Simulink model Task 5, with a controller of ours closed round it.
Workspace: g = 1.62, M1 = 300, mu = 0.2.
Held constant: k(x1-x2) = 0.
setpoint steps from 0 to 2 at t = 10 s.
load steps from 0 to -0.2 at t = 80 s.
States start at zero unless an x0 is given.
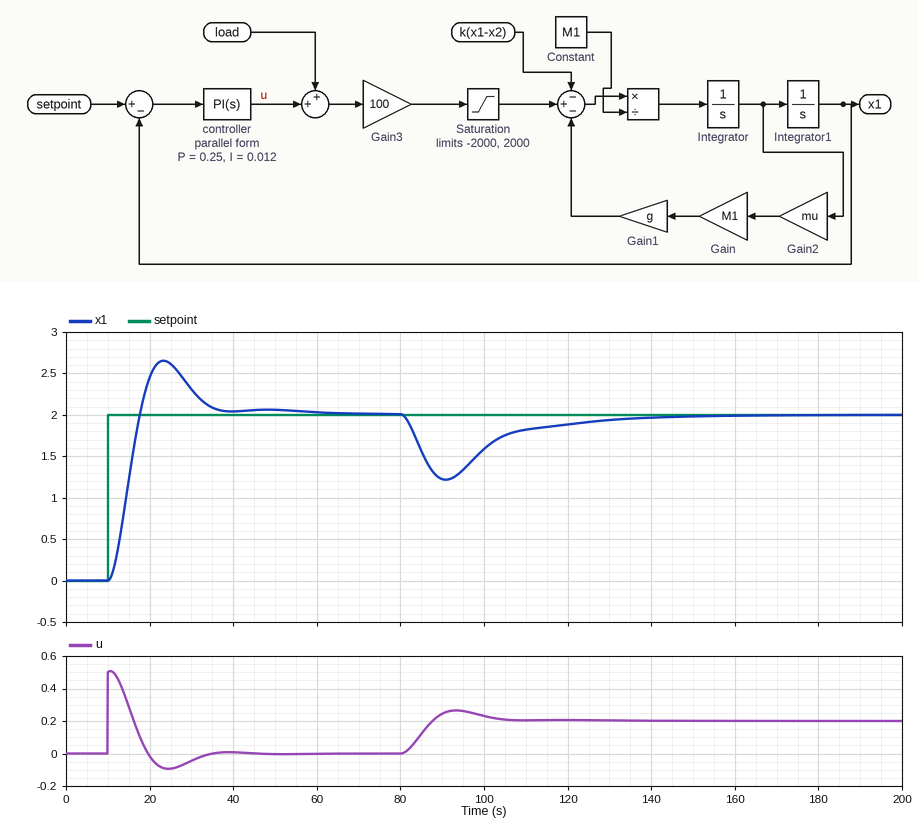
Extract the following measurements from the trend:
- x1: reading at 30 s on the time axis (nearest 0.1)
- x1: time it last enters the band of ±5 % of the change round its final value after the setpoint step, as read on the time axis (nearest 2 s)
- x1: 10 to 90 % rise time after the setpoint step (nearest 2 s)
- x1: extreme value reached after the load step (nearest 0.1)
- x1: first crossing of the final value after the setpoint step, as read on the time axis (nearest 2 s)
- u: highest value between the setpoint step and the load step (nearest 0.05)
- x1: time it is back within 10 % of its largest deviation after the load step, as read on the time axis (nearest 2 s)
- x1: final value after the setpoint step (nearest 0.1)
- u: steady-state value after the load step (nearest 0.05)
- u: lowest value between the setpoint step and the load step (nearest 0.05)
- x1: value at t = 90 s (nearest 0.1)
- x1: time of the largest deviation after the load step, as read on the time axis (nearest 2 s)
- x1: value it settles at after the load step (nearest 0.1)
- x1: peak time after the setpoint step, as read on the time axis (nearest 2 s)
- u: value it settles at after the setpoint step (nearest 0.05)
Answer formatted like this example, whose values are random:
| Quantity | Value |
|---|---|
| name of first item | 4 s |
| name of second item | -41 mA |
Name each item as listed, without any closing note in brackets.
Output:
| Quantity | Value |
|---|---|
| x1: reading at 30 s on the time axis | 2.3 |
| x1: time it last enters the band of ±5 % of the change round its final value after the setpoint step, as read on the time axis | 34 s |
| x1: 10 to 90 % rise time after the setpoint step | 6 s |
| x1: extreme value reached after the load step | 1.2 |
| x1: first crossing of the final value after the setpoint step, as read on the time axis | 18 s |
| u: highest value between the setpoint step and the load step | 0.50 |
| x1: time it is back within 10 % of its largest deviation after the load step, as read on the time axis | 126 s |
| x1: final value after the setpoint step | 2.0 |
| u: steady-state value after the load step | 0.20 |
| u: lowest value between the setpoint step and the load step | -0.10 |
| x1: value at t = 90 s | 1.2 |
| x1: time of the largest deviation after the load step, as read on the time axis | 90 s |
| x1: value it settles at after the load step | 2.0 |
| x1: peak time after the setpoint step, as read on the time axis | 24 s |
| u: value it settles at after the setpoint step | 0.00 |
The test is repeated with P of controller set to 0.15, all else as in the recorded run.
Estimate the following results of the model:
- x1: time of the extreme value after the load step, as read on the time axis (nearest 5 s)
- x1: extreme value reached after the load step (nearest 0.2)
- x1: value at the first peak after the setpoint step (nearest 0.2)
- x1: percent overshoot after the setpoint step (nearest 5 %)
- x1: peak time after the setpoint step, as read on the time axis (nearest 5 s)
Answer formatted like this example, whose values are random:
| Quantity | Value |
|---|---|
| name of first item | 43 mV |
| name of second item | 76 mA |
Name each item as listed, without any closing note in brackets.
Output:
| Quantity | Value |
|---|---|
| x1: time of the extreme value after the load step, as read on the time axis | 95 s |
| x1: extreme value reached after the load step | 1.0 |
| x1: value at the first peak after the setpoint step | 2.8 |
| x1: percent overshoot after the setpoint step | 45 % |
| x1: peak time after the setpoint step, as read on the time axis | 30 s |
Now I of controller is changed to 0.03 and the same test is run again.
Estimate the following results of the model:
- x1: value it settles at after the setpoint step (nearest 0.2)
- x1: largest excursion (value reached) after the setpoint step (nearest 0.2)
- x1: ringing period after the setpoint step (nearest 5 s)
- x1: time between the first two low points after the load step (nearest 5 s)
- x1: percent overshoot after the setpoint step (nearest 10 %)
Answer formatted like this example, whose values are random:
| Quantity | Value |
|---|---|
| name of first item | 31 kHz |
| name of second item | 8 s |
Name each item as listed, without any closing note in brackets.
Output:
| Quantity | Value |
|---|---|
| x1: value it settles at after the setpoint step | 2.0 |
| x1: largest excursion (value reached) after the setpoint step | 3.2 |
| x1: ringing period after the setpoint step | 30 s |
| x1: time between the first two low points after the load step | 30 s |
| x1: percent overshoot after the setpoint step | 60 % |
